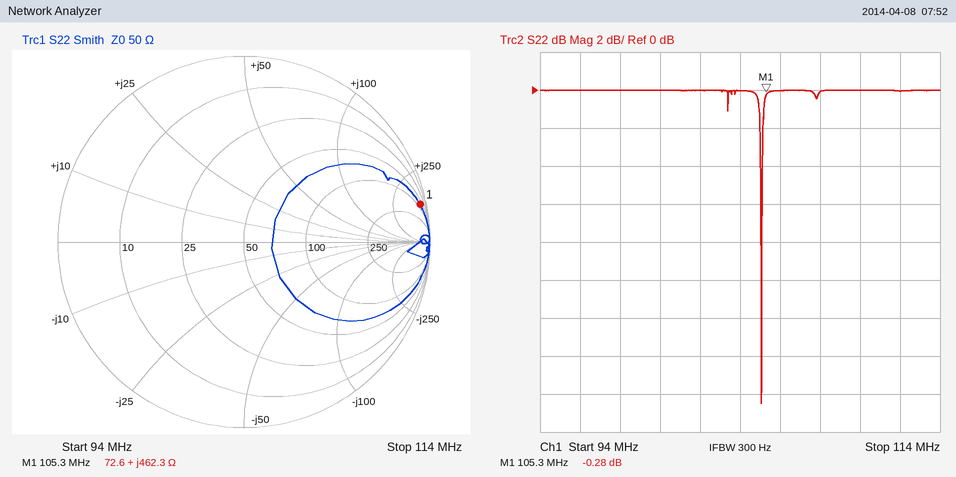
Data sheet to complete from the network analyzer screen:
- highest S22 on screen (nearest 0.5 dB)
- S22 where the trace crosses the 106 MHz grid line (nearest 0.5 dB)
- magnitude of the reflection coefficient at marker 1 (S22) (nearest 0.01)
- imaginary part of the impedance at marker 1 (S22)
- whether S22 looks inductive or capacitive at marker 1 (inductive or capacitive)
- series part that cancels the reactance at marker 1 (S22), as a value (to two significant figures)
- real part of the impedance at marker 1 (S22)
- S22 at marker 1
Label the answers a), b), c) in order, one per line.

a) 0.0 dB
b) 0.0 dB
c) 0.97
d) +462.3 Ω
e) inductive
f) 3.3 pF
g) 72.6 Ω
h) -0.28 dB
